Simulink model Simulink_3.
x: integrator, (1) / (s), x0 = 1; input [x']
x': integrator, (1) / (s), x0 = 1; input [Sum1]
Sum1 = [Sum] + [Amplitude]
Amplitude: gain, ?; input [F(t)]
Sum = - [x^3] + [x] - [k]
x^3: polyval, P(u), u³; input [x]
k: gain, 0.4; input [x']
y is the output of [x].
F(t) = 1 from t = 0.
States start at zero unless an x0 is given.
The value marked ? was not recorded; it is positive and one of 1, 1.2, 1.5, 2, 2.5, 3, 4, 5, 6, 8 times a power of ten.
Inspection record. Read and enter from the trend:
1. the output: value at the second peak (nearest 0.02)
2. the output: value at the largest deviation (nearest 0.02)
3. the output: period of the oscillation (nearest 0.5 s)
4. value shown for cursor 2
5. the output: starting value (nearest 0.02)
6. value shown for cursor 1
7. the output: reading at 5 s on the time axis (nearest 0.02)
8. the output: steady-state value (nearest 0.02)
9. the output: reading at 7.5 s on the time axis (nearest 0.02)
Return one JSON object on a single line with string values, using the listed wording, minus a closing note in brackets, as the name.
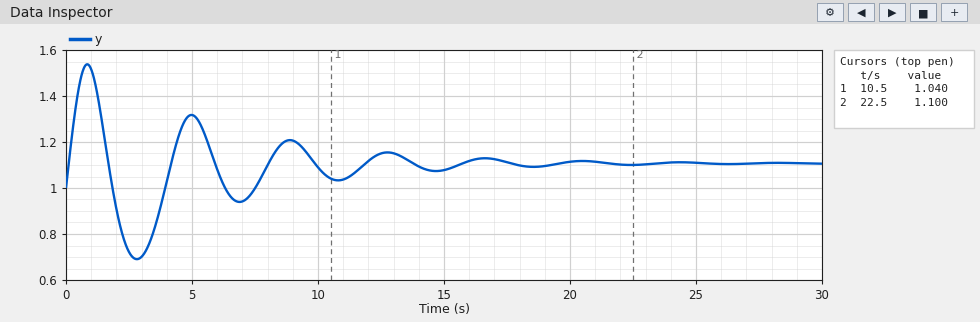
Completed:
{"the output: value at the second peak": "1.32", "the output: value at the largest deviation": "1.54", "the output: period of the oscillation": "4.0 s", "value shown for cursor 2": "1.100", "the output: starting value": "1.00", "value shown for cursor 1": "1.040", "the output: reading at 5 s on the time axis": "1.32", "the output: steady-state value": "1.10", "the output: reading at 7.5 s on the time axis": "1.00"}
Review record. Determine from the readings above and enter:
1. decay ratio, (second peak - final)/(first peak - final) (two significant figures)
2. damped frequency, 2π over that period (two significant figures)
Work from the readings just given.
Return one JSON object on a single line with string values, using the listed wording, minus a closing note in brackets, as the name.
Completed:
{"decay ratio, (second peak - final)/(first peak - final)": "0.50", "damped frequency, 2π over that period": "1.6 rad/s"}
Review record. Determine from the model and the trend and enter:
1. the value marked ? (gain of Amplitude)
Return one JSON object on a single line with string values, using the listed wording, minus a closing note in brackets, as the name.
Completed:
{"the value marked ?": "0.25"}
